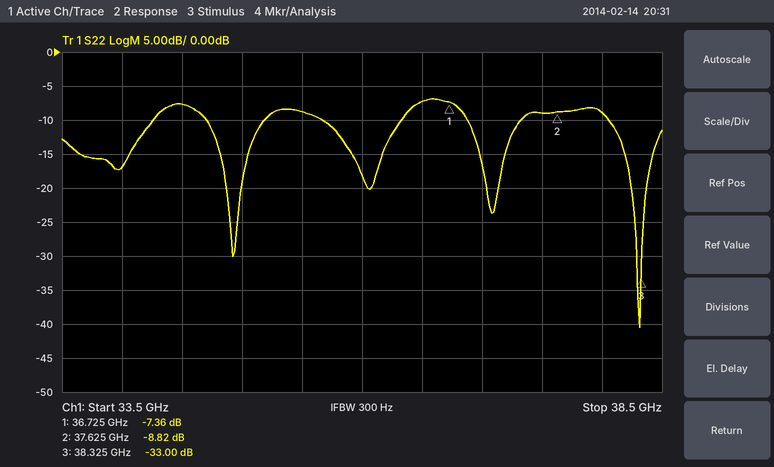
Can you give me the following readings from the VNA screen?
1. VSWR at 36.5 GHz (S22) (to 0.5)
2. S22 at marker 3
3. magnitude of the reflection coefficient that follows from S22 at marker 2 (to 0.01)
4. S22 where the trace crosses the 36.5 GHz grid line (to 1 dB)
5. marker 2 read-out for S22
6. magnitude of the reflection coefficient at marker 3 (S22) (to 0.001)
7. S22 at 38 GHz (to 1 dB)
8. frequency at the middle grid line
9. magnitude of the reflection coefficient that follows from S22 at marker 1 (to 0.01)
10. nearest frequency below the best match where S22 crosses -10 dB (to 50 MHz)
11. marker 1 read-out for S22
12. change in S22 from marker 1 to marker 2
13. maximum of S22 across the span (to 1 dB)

2.5
-33.00 dB
0.36
-7 dB
-8.82 dB
0.022
-9 dB
36 GHz
0.43
38.05 GHz
-7.36 dB
-1.46 dB
-7 dB
